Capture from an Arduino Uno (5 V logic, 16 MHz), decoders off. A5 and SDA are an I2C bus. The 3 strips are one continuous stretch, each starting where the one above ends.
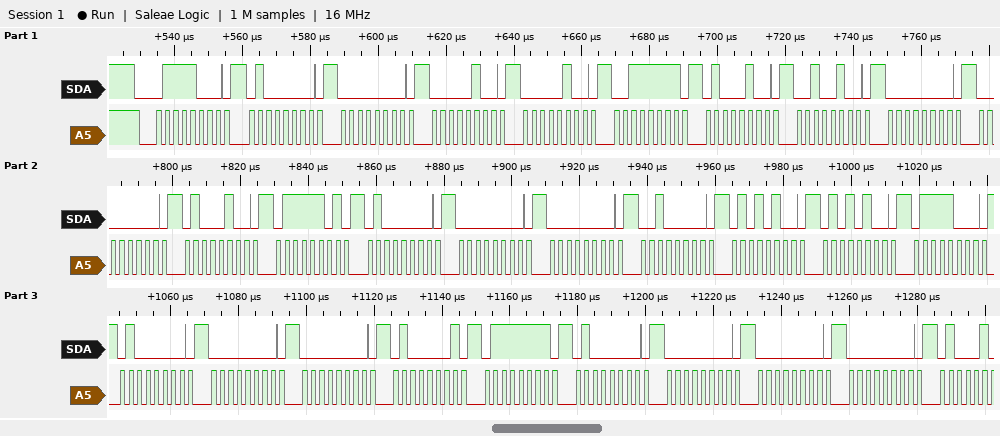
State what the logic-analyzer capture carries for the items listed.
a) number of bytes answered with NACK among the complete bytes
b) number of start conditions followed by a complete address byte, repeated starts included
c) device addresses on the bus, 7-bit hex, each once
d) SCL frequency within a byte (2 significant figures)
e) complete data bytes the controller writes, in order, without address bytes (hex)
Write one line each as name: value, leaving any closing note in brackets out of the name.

number of bytes answered with NACK among the complete bytes: 0
number of start conditions followed by a complete address byte, repeated starts included: 1
device addresses on the bus, 7-bit hex, each once: 0x3C
SCL frequency within a byte: 400 kHz
complete data bytes the controller writes, in order, without address bytes: 40 00 04 04 3F 44 24 00 00 44 7D 40 00 00 20 54 54 78 40 00 00 41 7F 40 00 00 00
